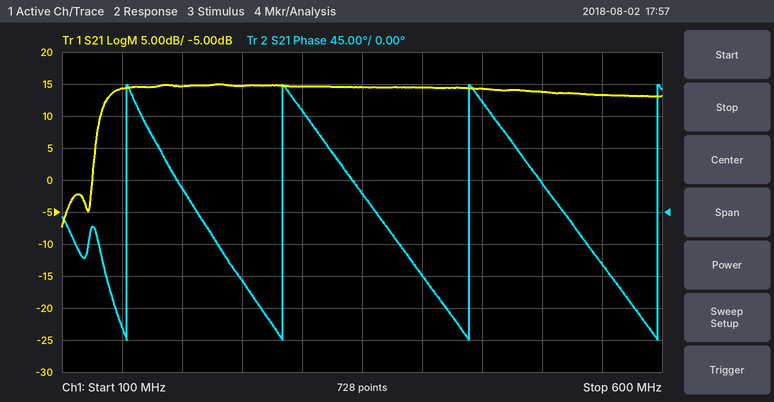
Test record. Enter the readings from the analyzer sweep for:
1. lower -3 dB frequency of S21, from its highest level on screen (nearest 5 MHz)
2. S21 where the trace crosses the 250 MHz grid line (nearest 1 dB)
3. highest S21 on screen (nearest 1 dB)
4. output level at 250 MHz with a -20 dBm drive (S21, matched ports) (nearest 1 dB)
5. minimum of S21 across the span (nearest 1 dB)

135 MHz
15 dB
15 dB
-5 dBm
-7 dB
